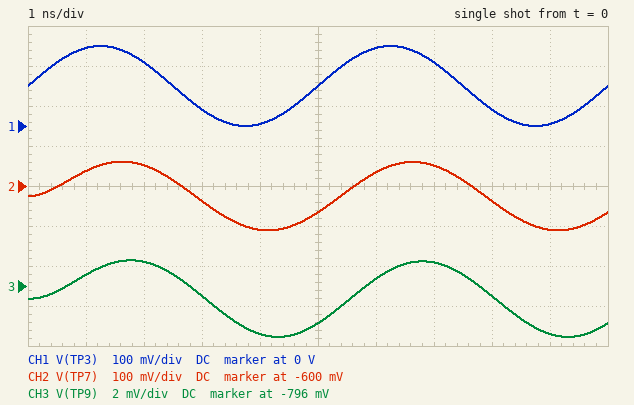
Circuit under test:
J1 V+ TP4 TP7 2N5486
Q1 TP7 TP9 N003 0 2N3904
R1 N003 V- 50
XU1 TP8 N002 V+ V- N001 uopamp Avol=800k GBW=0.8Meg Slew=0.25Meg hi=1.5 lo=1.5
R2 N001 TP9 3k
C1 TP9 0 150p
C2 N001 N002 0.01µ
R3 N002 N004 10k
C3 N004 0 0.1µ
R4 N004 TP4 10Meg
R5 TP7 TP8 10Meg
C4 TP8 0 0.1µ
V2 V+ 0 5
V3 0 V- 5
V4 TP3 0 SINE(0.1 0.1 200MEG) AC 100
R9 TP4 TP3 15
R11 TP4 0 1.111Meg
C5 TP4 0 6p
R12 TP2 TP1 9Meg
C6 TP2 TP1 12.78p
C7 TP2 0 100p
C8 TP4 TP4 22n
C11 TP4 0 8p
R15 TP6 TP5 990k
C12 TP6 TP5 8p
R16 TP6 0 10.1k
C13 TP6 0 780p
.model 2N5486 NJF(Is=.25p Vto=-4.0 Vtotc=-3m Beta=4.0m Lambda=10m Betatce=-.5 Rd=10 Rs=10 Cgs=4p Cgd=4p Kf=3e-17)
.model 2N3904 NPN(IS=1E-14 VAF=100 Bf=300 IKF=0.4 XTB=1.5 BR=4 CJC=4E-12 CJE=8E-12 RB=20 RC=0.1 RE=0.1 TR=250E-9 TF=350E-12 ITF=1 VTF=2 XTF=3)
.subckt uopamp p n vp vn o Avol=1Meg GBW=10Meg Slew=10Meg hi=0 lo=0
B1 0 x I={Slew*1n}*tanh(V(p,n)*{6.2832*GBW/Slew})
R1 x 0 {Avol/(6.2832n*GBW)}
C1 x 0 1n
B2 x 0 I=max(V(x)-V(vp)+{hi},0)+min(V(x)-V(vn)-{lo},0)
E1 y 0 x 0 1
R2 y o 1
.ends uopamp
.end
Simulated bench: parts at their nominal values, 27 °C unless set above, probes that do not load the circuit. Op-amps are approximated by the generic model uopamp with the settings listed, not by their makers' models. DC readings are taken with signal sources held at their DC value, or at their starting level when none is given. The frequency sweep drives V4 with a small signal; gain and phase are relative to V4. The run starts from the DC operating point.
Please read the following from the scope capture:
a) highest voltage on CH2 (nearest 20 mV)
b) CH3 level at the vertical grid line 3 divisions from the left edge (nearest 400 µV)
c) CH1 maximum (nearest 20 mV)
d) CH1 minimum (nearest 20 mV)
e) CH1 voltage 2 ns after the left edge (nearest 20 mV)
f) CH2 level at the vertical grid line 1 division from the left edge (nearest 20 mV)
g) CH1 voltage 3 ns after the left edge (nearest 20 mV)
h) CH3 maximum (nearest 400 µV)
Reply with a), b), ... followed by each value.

a) -540 mV
b) -796.4 mV
c) 200 mV
d) 0 V
e) 160 mV
f) -560 mV
g) 40 mV
h) -794.8 mV
